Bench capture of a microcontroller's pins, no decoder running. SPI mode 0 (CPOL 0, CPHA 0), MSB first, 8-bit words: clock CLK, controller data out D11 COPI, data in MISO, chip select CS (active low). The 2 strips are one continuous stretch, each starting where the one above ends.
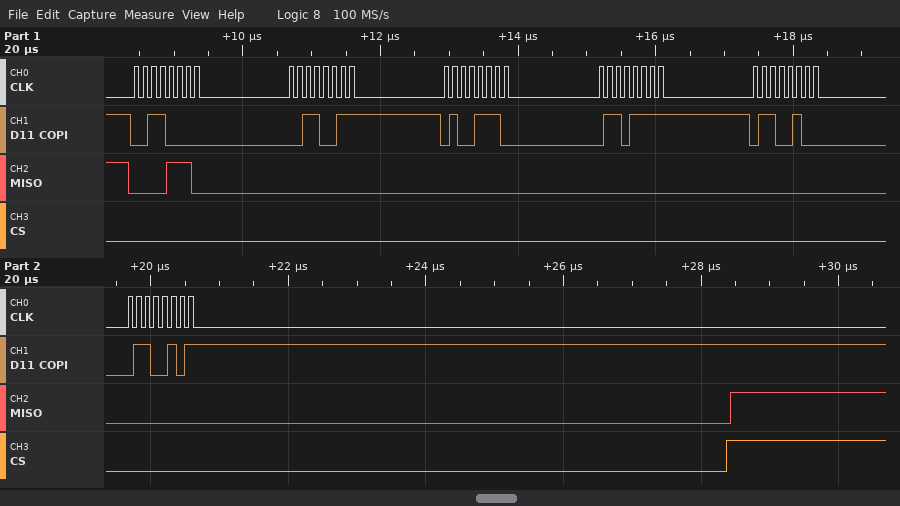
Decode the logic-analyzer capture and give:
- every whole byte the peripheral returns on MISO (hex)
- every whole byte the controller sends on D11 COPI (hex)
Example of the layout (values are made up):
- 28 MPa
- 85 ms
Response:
- 0E 00 00 00 00 00
- 30 33 4E 6F 64 65
